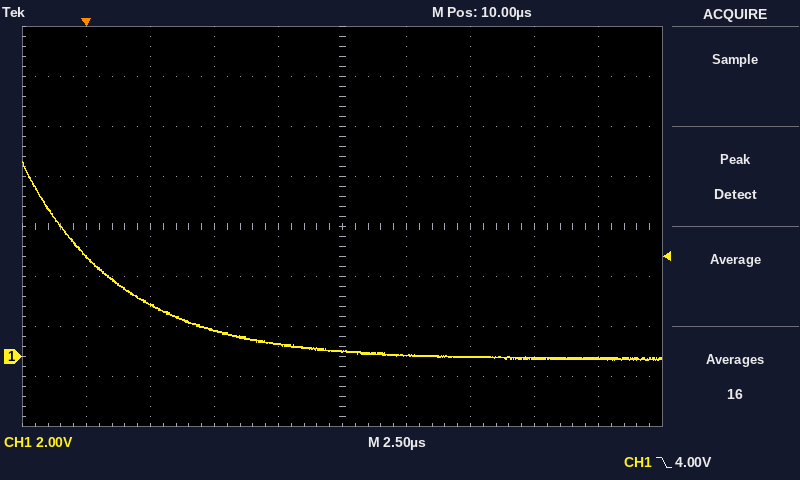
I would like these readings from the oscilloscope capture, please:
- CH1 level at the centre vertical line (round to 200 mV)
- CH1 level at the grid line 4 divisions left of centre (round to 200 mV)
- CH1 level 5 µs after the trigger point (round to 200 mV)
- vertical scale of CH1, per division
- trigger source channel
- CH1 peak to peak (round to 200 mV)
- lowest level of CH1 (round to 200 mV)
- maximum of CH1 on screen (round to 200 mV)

200 mV
4.0 V
1.0 V
2 V
CH1
8.0 V
-200 mV
7.8 V
